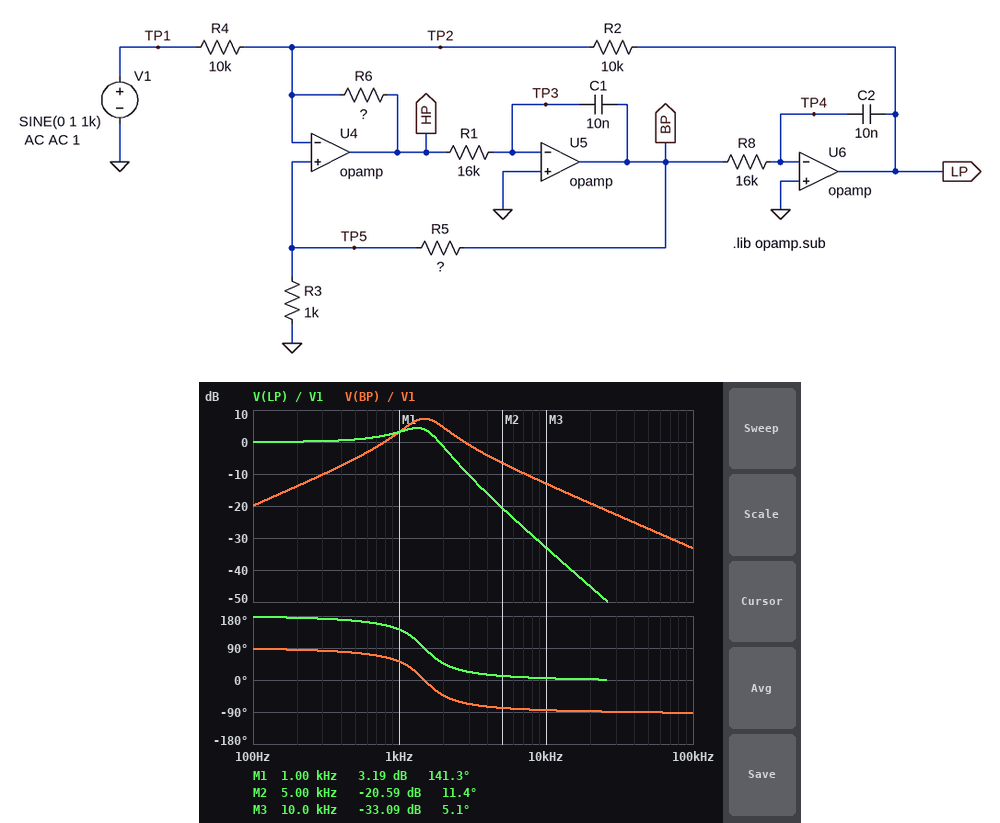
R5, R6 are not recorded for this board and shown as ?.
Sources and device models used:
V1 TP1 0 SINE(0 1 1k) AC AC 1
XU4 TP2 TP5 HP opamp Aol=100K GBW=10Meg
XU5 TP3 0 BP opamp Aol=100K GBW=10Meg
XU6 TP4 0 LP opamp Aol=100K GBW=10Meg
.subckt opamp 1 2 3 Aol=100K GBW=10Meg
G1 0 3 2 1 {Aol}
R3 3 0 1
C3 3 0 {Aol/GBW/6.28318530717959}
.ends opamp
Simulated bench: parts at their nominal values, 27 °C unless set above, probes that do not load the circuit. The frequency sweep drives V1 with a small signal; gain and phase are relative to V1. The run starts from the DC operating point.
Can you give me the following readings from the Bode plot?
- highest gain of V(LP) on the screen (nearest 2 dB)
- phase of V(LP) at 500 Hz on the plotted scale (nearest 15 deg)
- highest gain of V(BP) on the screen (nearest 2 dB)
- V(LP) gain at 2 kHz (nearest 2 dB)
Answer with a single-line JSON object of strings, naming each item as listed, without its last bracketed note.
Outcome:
{"highest gain of V(LP) on the screen": "4 dB", "phase of V(LP) at 500 Hz on the plotted scale": "165 deg", "highest gain of V(BP) on the screen": "8 dB", "V(LP) gain at 2 kHz": "-2 dB"}
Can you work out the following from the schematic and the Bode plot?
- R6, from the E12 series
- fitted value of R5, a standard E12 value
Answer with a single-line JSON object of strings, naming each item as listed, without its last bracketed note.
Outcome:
{"R6, from the E12 series": "22 kΩ", "fitted value of R5, a standard E12 value": "4.7 kΩ"}
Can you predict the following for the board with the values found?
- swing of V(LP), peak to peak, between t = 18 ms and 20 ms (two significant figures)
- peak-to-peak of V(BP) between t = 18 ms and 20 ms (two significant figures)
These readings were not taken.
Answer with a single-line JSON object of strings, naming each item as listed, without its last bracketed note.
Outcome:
{"swing of V(LP), peak to peak, between t = 18 ms and 20 ms": "2.9 V", "peak-to-peak of V(BP) between t = 18 ms and 20 ms": "2.9 V"}
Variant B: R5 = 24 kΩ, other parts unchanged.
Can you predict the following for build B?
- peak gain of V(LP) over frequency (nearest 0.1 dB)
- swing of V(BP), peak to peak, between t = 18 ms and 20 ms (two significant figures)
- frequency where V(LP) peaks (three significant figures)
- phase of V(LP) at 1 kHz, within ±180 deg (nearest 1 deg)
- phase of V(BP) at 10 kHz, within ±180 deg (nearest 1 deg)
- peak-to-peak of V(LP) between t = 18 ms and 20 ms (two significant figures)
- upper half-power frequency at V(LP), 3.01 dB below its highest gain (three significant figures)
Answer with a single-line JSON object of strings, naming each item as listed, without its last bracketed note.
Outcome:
{"peak gain of V(LP) over frequency": "16.8 dB", "swing of V(BP), peak to peak, between t = 18 ms and 20 ms": "3.7 V", "frequency where V(LP) peaks": "1.47 kHz", "phase of V(LP) at 1 kHz, within ±180 deg": "170 deg", "phase of V(BP) at 10 kHz, within ±180 deg": "-89 deg", "peak-to-peak of V(LP) between t = 18 ms and 20 ms": "3.6 V", "upper half-power frequency at V(LP), 3.01 dB below its highest gain": "1.57 kHz"}
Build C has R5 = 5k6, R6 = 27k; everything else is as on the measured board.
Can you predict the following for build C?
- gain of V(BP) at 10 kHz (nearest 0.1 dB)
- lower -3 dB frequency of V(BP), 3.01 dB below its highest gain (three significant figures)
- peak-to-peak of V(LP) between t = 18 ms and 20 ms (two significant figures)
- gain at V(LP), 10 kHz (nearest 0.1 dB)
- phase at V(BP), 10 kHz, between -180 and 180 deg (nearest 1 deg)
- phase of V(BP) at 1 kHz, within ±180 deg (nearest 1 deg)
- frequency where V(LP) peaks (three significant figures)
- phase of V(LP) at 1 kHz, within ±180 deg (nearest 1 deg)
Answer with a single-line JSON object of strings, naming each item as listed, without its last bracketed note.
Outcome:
{"gain of V(BP) at 10 kHz": "-11.2 dB", "lower -3 dB frequency of V(BP), 3.01 dB below its highest gain": "1.22 kHz", "peak-to-peak of V(LP) between t = 18 ms and 20 ms": "2.8 V", "gain at V(LP), 10 kHz": "-31.3 dB", "phase at V(BP), 10 kHz, between -180 and 180 deg": "-85 deg", "phase of V(BP) at 1 kHz, within ±180 deg": "60 deg", "frequency where V(LP) peaks": "1.49 kHz", "phase of V(LP) at 1 kHz, within ±180 deg": "150 deg"}
